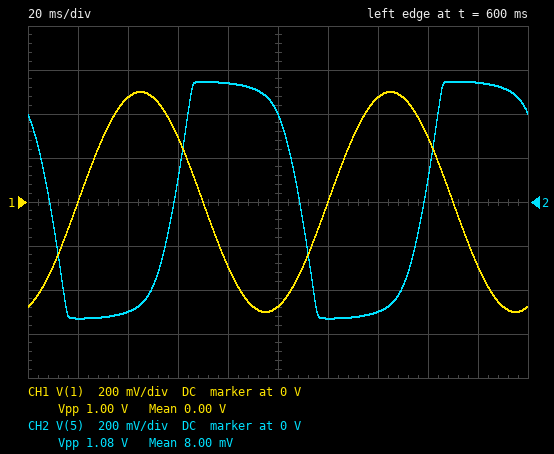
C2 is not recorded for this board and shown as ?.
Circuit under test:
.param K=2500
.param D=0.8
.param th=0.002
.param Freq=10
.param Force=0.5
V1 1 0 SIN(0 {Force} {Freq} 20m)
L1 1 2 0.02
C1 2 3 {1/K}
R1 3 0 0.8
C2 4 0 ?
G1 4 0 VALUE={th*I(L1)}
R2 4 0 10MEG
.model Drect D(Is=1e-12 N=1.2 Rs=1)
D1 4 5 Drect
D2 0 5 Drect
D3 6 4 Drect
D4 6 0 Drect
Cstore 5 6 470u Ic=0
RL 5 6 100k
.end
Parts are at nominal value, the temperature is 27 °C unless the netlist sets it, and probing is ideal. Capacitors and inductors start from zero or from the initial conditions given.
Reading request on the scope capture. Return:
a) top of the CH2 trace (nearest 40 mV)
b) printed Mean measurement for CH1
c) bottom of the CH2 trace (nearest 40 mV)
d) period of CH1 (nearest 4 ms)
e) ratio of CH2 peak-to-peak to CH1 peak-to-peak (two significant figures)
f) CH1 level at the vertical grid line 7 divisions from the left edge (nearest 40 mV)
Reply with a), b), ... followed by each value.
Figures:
a) 560 mV
b) 0.00 V
c) -520 mV
d) 100 ms
e) 1.1
f) 480 mV
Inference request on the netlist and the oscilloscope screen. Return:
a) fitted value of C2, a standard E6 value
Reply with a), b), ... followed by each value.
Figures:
a) 150 nF
